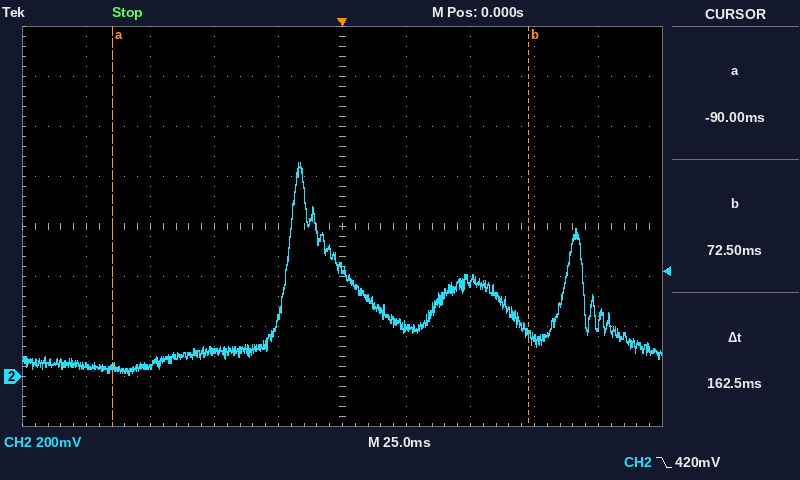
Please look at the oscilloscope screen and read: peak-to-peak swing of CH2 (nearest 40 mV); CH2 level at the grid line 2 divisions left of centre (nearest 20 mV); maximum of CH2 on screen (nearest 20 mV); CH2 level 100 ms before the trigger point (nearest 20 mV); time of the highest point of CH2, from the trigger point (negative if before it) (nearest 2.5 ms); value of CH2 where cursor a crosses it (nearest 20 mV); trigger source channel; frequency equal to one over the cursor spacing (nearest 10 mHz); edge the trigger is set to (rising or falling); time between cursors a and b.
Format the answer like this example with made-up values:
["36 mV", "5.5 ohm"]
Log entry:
["840 mV", "100 mV", "860 mV", "40 mV", "-17.5 ms", "40 mV", "CH2", "6.15 Hz", "falling", "162.5 ms"]
